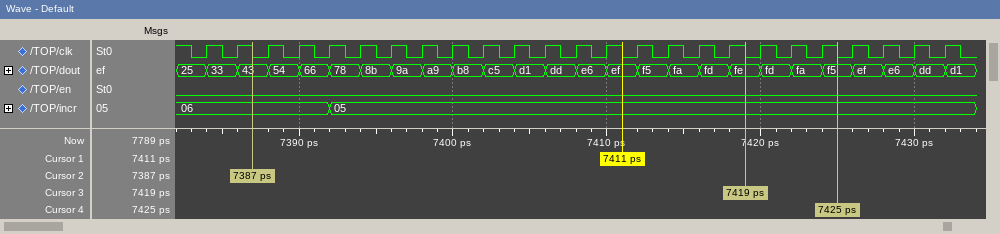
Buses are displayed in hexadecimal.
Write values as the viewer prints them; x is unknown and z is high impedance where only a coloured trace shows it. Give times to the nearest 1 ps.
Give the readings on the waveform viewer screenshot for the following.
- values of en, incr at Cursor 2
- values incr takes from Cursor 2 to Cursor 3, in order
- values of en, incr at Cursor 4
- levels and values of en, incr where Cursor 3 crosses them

en=0, incr=06
06, 05
en=0, incr=05
en=0, incr=05
